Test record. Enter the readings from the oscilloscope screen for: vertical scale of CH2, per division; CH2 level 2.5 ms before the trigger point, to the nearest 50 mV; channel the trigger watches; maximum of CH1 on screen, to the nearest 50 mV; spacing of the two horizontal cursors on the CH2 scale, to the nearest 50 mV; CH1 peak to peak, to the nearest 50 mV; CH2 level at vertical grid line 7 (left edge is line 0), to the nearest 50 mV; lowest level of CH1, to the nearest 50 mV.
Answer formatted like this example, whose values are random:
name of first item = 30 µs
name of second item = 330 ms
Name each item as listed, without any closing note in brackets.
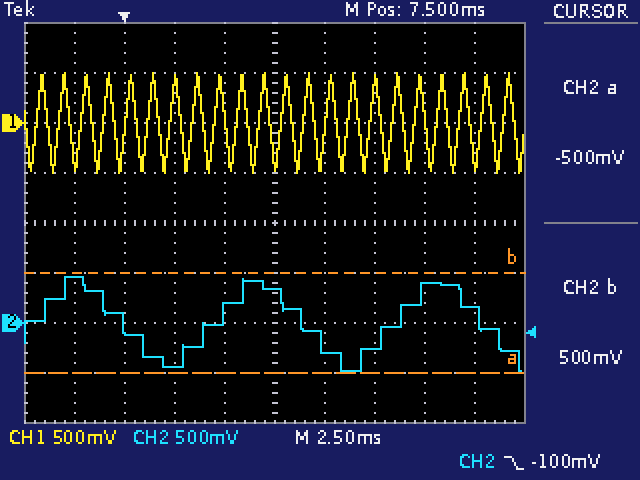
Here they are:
vertical scale of CH2, per division = 500 mV
CH2 level 2.5 ms before the trigger point, to the nearest 50 mV = 450 mV
channel the trigger watches = CH2
maximum of CH1 on screen, to the nearest 50 mV = 500 mV
spacing of the two horizontal cursors on the CH2 scale, to the nearest 50 mV = 1.00 V
CH1 peak to peak, to the nearest 50 mV = 1.00 V
CH2 level at vertical grid line 7 (left edge is line 0), to the nearest 50 mV = -250 mV
lowest level of CH1, to the nearest 50 mV = -500 mV
